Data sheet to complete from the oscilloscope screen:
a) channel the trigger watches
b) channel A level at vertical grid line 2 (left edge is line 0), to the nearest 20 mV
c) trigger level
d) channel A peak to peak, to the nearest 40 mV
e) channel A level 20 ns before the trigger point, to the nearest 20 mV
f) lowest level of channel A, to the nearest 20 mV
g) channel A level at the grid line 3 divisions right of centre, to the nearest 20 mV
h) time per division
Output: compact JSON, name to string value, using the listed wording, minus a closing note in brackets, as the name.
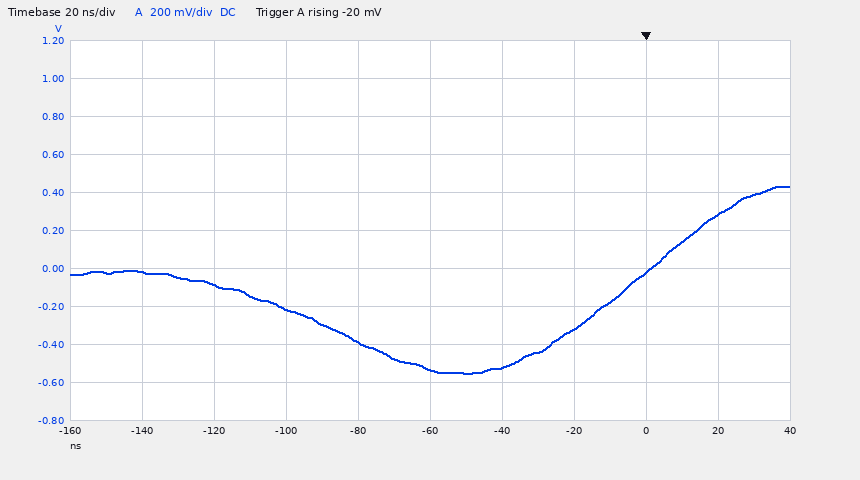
{"channel the trigger watches": "channel A", "channel A level at vertical grid line 2 (left edge is line 0), to the nearest 20 mV": "-80 mV", "trigger level": "-20 mV", "channel A peak to peak, to the nearest 40 mV": "1.00 V", "channel A level 20 ns before the trigger point, to the nearest 20 mV": "-320 mV", "lowest level of channel A, to the nearest 20 mV": "-560 mV", "channel A level at the grid line 3 divisions right of centre, to the nearest 20 mV": "-20 mV", "time per division": "20 ns"}
